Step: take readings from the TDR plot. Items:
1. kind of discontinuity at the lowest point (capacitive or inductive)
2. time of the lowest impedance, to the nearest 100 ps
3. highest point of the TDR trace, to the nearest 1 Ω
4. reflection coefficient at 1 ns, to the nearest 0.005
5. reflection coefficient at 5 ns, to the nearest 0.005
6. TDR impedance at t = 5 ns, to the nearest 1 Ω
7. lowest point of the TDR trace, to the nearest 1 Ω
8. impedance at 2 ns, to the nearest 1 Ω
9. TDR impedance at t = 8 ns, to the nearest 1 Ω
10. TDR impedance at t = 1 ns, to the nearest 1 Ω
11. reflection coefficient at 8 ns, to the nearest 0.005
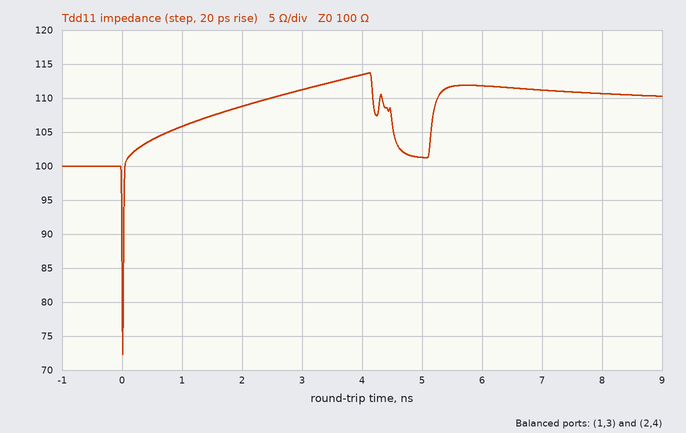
capacitive
0.0 ns
114 Ω
+0.030
+0.005
101 Ω
72 Ω
109 Ω
111 Ω
106 Ω
+0.050
